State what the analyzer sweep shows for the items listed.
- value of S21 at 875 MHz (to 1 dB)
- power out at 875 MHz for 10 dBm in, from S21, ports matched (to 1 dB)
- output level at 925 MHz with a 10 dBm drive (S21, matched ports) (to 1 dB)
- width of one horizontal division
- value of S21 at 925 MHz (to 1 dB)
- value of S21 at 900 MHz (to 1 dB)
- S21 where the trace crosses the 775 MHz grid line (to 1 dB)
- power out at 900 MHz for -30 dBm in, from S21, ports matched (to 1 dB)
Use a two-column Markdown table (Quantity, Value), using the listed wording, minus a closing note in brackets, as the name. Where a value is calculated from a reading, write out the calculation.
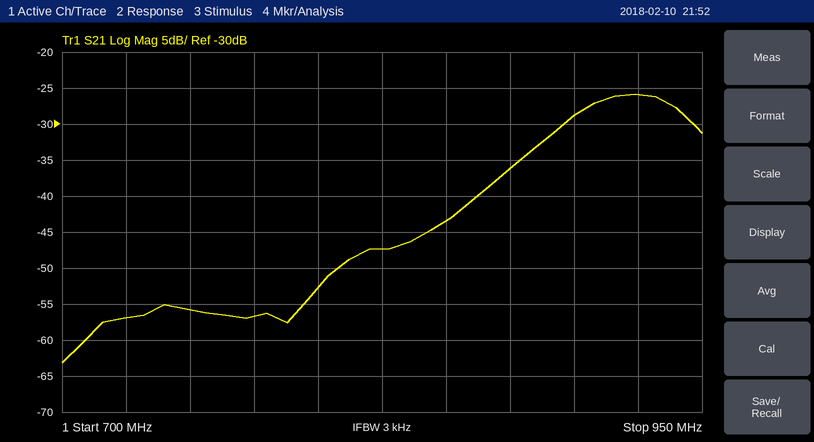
| Quantity | Value |
|---|---|
| value of S21 at 875 MHz | -36 dB |
| power out at 875 MHz for 10 dBm in, from S21, ports matched | 10 dBm + (-36 dB) = -26 dBm |
| output level at 925 MHz with a 10 dBm drive (S21, matched ports) | 10 dBm + (-26 dB) = -16 dBm |
| width of one horizontal division | 25 MHz |
| value of S21 at 925 MHz | -26 dB |
| value of S21 at 900 MHz | -29 dB |
| S21 where the trace crosses the 775 MHz grid line | -57 dB |
| power out at 900 MHz for -30 dBm in, from S21, ports matched | -30 dBm + (-29 dB) = -59 dBm |
